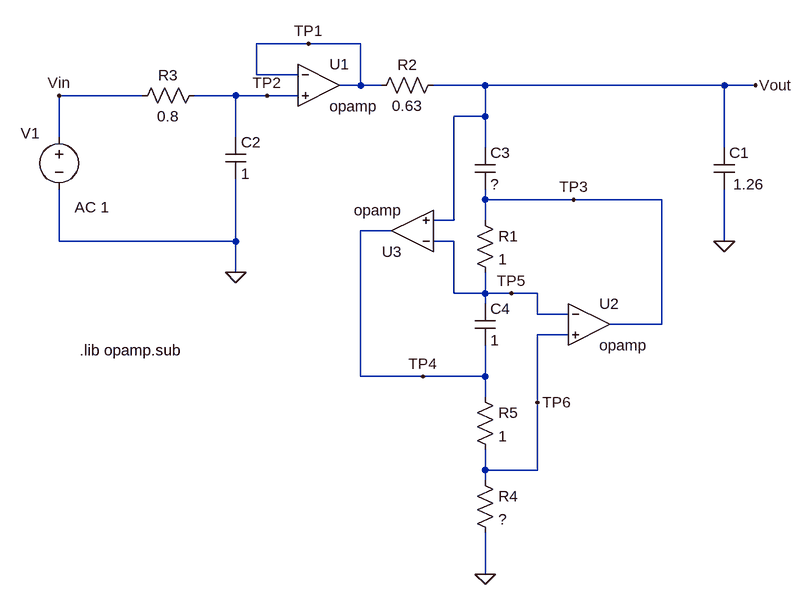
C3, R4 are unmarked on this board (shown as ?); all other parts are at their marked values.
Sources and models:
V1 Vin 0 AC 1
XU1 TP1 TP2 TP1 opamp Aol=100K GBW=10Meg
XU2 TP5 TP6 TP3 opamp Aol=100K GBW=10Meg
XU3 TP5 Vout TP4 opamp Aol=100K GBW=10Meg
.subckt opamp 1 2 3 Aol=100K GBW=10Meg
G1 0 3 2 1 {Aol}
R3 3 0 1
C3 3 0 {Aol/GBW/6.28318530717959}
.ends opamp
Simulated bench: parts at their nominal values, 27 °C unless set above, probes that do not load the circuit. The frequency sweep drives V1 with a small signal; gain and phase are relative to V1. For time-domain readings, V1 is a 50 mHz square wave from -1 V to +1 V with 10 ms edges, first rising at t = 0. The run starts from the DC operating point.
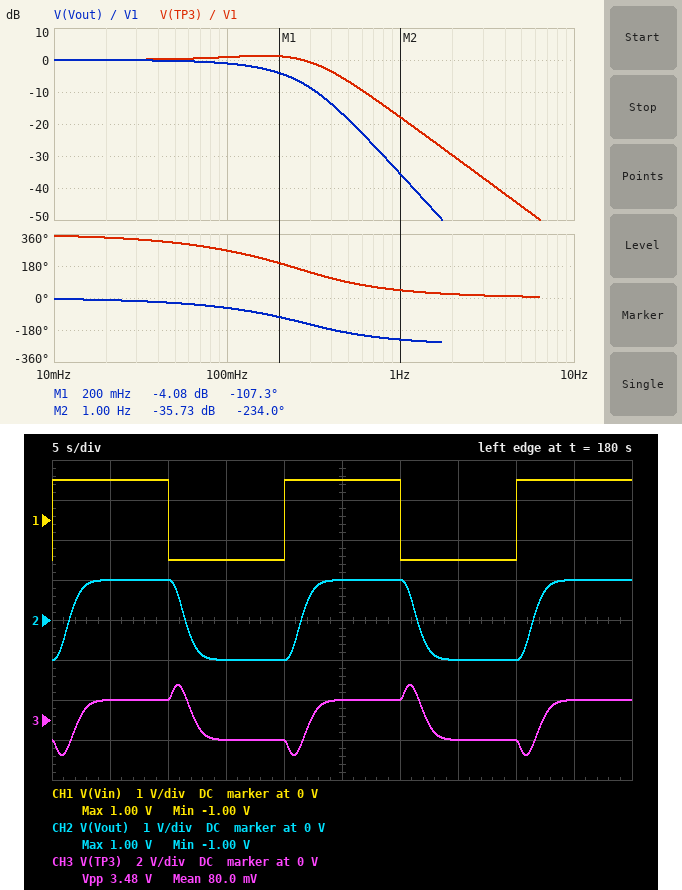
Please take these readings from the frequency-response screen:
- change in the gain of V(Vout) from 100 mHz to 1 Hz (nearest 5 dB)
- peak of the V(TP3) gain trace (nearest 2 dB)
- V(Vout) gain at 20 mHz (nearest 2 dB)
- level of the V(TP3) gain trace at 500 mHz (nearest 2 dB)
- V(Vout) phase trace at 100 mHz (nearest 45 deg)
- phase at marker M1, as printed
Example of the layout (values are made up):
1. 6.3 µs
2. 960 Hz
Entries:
1. -35 dB
2. 2 dB
3. 0 dB
4. -6 dB
5. -45 deg
6. -107.3 deg
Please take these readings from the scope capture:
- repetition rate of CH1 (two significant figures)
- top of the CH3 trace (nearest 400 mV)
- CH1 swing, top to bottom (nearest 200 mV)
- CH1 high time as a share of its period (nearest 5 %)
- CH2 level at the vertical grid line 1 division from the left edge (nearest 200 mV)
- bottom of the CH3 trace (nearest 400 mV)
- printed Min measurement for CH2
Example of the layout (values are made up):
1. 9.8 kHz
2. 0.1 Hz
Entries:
1. 50 mHz
2. 1.6 V
3. 2.0 V
4. 50 %
5. 1.0 V
6. -1.6 V
7. -1.00 V
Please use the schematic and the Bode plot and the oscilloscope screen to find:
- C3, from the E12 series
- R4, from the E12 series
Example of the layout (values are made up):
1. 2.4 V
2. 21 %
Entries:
1. 390 mF
2. 0.82 Ω
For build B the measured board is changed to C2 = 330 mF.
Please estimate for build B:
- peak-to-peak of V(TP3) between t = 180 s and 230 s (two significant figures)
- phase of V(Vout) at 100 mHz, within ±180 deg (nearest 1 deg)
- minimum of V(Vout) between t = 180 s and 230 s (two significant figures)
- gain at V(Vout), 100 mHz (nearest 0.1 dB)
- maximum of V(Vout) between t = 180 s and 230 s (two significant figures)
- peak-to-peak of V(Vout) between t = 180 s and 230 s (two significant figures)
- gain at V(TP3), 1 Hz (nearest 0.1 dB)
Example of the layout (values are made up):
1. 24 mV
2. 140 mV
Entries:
1. 4.4 V
2. -39 deg
3. -1.1 V
4. -0.2 dB
5. 1.1 V
6. 2.1 V
7. -9.5 dB
